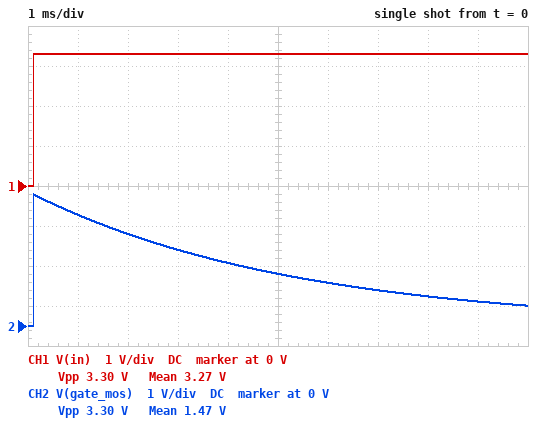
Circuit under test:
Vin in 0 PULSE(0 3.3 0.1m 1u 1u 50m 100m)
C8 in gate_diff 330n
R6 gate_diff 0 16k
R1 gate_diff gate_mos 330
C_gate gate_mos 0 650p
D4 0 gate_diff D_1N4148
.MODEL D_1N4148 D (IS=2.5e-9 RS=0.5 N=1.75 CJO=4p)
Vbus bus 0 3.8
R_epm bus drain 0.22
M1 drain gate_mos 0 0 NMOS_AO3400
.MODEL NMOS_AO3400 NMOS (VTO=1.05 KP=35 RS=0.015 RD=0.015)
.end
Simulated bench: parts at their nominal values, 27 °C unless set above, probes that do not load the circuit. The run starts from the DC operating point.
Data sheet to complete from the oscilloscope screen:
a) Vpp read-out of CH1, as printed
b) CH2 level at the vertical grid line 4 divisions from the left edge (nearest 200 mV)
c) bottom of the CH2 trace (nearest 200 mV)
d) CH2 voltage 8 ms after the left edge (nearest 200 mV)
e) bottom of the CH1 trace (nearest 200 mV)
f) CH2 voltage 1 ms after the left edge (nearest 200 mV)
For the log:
3.30 V
1.6 V
0 V
800 mV
0 V
2.8 V
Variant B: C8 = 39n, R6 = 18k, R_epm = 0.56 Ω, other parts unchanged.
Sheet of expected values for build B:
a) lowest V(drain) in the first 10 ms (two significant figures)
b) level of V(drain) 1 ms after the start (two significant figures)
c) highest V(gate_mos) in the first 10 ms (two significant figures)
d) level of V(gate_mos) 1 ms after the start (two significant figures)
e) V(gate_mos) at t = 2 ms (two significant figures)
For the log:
280 mV
3.8 V
3.2 V
920 mV
230 mV
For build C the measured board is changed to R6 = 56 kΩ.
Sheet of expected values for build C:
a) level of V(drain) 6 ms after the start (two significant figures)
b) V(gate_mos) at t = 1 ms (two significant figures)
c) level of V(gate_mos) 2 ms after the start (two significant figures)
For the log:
820 mV
3.1 V
3.0 V
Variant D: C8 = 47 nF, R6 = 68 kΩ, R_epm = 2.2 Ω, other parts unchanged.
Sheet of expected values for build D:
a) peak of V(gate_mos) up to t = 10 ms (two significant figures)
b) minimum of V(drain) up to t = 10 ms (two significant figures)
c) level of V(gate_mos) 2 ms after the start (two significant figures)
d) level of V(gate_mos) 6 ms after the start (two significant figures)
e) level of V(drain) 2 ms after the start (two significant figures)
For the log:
3.3 V
73 mV
1.8 V
530 mV
120 mV
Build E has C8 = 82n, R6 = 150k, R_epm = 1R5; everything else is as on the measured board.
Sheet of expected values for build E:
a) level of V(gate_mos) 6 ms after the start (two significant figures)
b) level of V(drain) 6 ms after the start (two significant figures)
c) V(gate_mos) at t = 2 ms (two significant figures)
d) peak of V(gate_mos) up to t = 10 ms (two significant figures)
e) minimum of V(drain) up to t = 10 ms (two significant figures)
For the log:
2.0 V
150 mV
2.8 V
3.3 V
110 mV
